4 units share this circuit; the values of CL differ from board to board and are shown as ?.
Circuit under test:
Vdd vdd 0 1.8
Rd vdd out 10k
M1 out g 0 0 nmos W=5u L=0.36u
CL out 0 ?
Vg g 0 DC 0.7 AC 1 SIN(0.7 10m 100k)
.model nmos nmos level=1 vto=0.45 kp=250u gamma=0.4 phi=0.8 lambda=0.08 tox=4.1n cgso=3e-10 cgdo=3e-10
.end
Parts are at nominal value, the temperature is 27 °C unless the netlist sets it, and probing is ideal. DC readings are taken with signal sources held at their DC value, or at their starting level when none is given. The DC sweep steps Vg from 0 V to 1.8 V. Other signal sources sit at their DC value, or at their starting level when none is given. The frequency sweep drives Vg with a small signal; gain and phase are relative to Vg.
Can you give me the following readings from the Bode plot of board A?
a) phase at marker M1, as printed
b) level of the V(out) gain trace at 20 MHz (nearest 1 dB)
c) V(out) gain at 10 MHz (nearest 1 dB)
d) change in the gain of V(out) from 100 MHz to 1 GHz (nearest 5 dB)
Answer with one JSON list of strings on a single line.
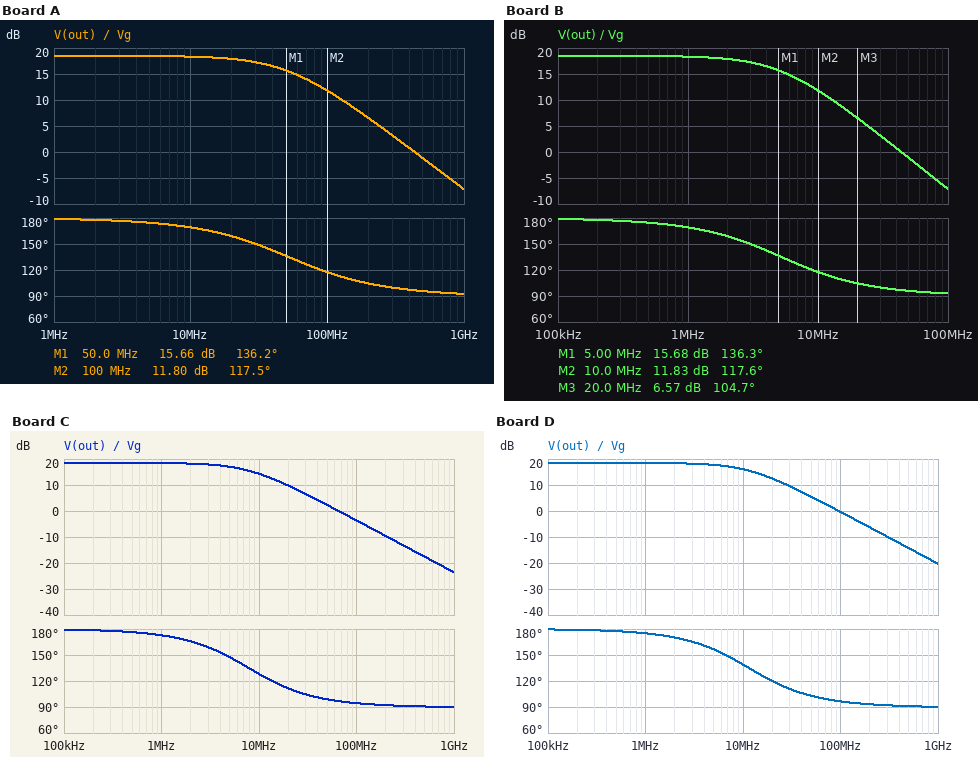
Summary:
["136.2 deg", "18 dB", "18 dB", "-20 dB"]
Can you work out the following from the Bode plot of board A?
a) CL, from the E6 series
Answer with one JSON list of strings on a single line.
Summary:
["330 fF"]
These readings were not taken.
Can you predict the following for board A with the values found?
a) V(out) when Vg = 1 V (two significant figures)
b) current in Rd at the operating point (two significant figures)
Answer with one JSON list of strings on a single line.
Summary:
["97 mV", "110 µA"]
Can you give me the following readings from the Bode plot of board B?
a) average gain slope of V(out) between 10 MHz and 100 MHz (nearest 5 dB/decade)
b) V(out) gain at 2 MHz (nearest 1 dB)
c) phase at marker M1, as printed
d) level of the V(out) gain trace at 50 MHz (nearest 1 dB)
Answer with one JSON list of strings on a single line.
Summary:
["-20 dB/decade", "18 dB", "136.3 deg", "-1 dB"]
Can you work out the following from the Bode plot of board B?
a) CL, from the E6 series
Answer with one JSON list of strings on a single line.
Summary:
["3.3 pF"]
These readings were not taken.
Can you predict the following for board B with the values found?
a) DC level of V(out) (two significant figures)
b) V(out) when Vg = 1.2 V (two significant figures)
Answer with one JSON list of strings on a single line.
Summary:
["660 mV", "69 mV"]
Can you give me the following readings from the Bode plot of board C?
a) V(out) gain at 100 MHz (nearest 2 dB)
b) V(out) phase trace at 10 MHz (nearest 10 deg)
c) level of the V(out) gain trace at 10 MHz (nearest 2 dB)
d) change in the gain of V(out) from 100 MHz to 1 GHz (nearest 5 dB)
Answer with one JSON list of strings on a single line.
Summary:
["-4 dB", "130 deg", "14 dB", "-20 dB"]
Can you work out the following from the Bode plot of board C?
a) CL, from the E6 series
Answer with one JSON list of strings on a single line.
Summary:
["2.2 pF"]
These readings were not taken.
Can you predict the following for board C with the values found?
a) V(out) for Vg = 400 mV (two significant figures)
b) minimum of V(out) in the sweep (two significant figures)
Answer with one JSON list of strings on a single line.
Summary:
["1.8 V", "38 mV"]
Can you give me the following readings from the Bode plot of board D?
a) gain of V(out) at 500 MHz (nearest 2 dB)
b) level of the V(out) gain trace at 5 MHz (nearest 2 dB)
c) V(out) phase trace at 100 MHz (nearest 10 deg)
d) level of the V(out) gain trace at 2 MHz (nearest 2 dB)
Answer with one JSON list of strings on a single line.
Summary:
["-14 dB", "18 dB", "100 deg", "18 dB"]
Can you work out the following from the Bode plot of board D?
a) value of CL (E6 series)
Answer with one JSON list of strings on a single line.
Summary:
["1.5 pF"]
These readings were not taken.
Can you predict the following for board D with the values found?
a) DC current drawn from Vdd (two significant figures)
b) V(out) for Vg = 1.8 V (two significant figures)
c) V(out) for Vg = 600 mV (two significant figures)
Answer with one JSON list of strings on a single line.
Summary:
["110 µA", "38 mV", "1.4 V"]
